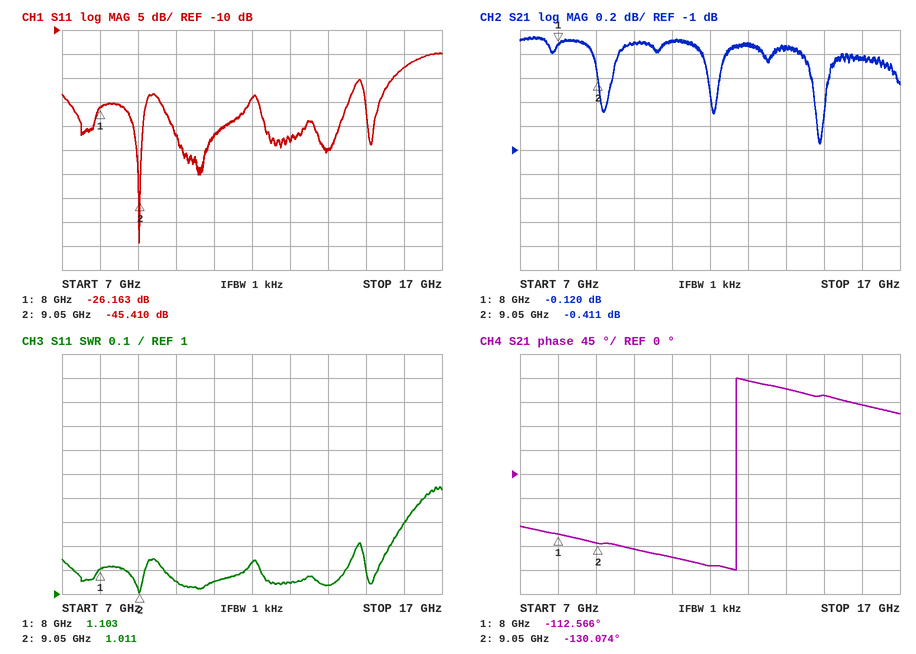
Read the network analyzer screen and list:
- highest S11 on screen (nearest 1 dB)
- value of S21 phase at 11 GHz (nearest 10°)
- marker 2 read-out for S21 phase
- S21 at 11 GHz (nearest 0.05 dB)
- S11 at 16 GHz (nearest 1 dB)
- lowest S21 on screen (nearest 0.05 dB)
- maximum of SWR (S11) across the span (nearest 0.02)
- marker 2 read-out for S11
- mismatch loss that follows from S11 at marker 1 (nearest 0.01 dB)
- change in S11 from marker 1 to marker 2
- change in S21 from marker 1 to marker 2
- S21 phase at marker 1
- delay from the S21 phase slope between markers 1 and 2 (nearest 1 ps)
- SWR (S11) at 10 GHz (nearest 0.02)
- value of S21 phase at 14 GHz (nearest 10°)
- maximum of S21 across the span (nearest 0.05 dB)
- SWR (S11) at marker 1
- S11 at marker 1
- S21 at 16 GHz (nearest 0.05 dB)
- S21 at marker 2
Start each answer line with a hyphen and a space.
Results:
- -15 dB
- -160°
- -130.074°
- -0.10 dB
- -18 dB
- -0.95 dB
- 1.44
- -45.410 dB
- 0.01 dB
- -19.247 dB
- -0.291 dB
- -112.566°
- 46 ps
- 1.06
- 160°
- -0.05 dB
- 1.103
- -26.163 dB
- -0.25 dB
- -0.411 dB
